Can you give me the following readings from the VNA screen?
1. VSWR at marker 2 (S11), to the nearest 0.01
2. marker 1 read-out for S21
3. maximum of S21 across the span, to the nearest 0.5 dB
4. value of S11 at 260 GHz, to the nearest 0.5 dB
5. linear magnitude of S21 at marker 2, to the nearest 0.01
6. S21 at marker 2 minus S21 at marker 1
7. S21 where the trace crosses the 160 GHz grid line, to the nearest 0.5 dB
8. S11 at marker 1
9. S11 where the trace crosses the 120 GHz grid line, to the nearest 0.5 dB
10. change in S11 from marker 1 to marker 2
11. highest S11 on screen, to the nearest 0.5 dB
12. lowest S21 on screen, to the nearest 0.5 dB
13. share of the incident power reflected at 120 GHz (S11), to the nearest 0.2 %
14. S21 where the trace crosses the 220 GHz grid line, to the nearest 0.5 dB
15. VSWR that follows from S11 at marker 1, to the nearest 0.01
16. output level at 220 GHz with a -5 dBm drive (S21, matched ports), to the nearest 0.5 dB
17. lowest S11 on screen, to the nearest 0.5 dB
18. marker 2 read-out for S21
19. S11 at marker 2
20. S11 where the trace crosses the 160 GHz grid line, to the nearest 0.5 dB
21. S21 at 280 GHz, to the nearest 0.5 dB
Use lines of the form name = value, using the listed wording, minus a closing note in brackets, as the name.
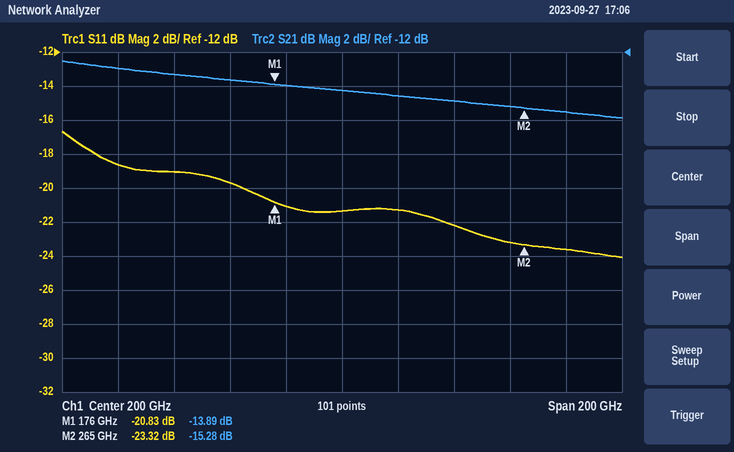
VSWR at marker 2 (S11), to the nearest 0.01 = 1.15
marker 1 read-out for S21 = -13.89 dB
maximum of S21 across the span, to the nearest 0.5 dB = -12.5 dB
value of S11 at 260 GHz, to the nearest 0.5 dB = -23.0 dB
linear magnitude of S21 at marker 2, to the nearest 0.01 = 0.17
S21 at marker 2 minus S21 at marker 1 = -1.39 dB
S21 where the trace crosses the 160 GHz grid line, to the nearest 0.5 dB = -13.5 dB
S11 at marker 1 = -20.83 dB
S11 where the trace crosses the 120 GHz grid line, to the nearest 0.5 dB = -18.5 dB
change in S11 from marker 1 to marker 2 = -2.49 dB
highest S11 on screen, to the nearest 0.5 dB = -16.5 dB
lowest S21 on screen, to the nearest 0.5 dB = -16.0 dB
share of the incident power reflected at 120 GHz (S11), to the nearest 0.2 % = 1.4 %
S21 where the trace crosses the 220 GHz grid line, to the nearest 0.5 dB = -14.5 dB
VSWR that follows from S11 at marker 1, to the nearest 0.01 = 1.20
output level at 220 GHz with a -5 dBm drive (S21, matched ports), to the nearest 0.5 dB = -19.5 dBm
lowest S11 on screen, to the nearest 0.5 dB = -24.0 dB
marker 2 read-out for S21 = -15.28 dB
S11 at marker 2 = -23.32 dB
S11 where the trace crosses the 160 GHz grid line, to the nearest 0.5 dB = -19.5 dB
S21 at 280 GHz, to the nearest 0.5 dB = -15.5 dB
